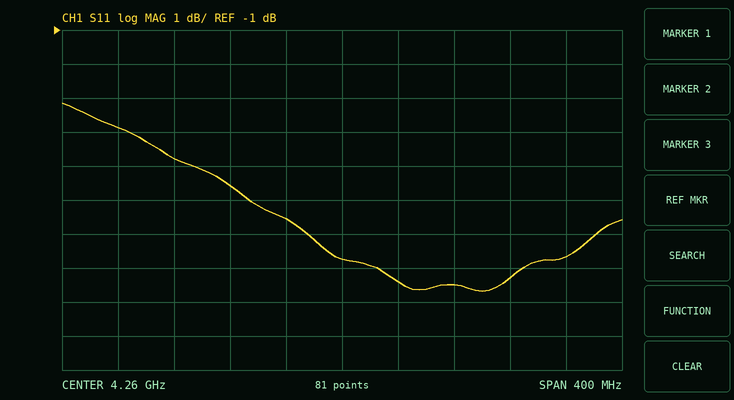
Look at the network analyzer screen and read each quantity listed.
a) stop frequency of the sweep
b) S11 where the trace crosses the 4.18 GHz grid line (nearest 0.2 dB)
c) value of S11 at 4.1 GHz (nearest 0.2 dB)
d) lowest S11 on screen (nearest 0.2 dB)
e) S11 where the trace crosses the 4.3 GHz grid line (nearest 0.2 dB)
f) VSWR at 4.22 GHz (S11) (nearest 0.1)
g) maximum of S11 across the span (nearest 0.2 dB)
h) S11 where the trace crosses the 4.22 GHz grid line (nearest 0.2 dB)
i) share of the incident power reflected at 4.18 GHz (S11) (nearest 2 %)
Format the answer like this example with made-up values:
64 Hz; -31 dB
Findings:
4.46 GHz; -5.6 dB; -3.8 dB; -8.6 dB; -8.4 dB; 2.8; -3.2 dB; -6.6 dB; 28 %
